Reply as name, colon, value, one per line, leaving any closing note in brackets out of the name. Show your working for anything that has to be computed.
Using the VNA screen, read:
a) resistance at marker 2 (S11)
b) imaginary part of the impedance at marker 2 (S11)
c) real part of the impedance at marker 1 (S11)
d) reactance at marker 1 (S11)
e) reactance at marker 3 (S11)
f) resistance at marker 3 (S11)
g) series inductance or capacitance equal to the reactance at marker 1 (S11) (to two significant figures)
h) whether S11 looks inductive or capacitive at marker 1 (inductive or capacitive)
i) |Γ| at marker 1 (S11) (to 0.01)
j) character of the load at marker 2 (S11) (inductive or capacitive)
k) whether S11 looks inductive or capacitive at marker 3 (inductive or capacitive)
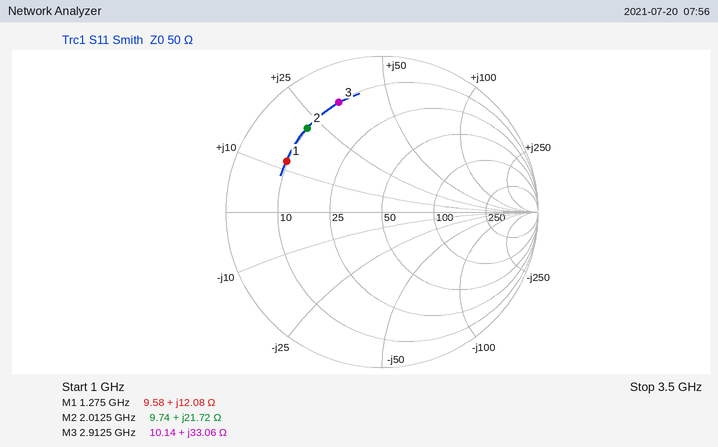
resistance at marker 2: 9.74 Ω
imaginary part of the impedance at marker 2: +21.72 Ω
real part of the impedance at marker 1: 9.58 Ω
reactance at marker 1: +12.08 Ω
reactance at marker 3: +33.06 Ω
resistance at marker 3: 10.14 Ω
series inductance or capacitance equal to the reactance at marker 1 (S11): L = 12.08 Ω/(2π × 1.275 GHz) ≈ 1.5 nH
whether S11 looks inductive or capacitive at marker 1: inductive
|Γ| at marker 1 (S11): 0.69
character of the load at marker 2 (S11): inductive
whether S11 looks inductive or capacitive at marker 3: inductive
